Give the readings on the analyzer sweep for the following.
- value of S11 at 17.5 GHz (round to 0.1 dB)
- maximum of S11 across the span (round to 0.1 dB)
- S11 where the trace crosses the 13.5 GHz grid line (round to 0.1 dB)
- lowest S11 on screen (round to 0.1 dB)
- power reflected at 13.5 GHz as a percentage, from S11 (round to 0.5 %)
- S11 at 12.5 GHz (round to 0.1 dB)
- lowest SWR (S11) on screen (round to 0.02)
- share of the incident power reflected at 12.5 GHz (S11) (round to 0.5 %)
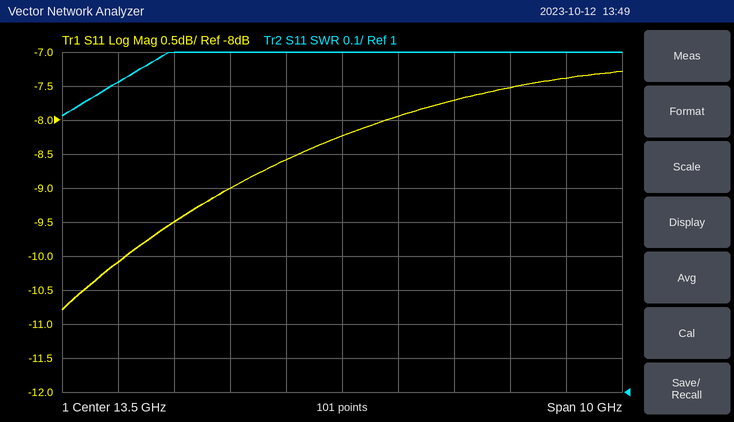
-7.4 dB
-7.3 dB
-8.2 dB
-10.8 dB
15.0 %
-8.6 dB
1.82
14.0 %
